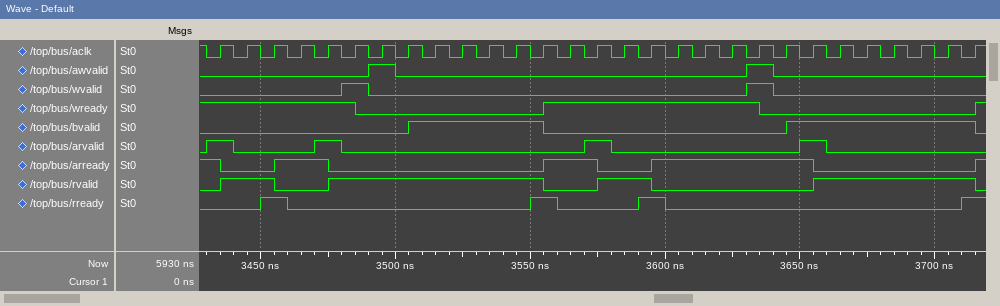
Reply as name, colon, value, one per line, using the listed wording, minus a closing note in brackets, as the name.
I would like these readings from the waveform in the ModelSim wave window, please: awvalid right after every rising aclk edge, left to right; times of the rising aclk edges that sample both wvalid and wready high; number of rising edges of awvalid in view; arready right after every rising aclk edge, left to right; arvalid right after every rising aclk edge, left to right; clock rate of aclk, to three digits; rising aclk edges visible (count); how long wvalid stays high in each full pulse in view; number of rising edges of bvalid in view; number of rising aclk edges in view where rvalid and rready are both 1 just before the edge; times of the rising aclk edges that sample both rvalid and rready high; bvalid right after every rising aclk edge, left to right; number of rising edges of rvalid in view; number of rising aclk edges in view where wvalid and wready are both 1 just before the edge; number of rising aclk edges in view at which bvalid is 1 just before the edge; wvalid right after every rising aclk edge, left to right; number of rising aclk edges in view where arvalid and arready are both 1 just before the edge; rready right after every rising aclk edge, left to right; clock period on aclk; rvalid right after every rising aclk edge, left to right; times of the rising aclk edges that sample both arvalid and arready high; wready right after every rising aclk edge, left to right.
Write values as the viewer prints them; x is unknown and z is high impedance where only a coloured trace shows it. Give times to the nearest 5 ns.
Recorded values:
awvalid right after every rising aclk edge, left to right: 0 0 0 0 0 0 1 0 0 0 0 0 0 0 0 0 0 0 0 0 1 0 0 0 0 0 0 0 0
times of the rising aclk edges that sample both wvalid and wready high: 3485 ns, 3635 ns
number of rising edges of awvalid in view: 2
arready right after every rising aclk edge, left to right: 0 0 1 1 0 0 0 0 0 0 0 0 1 1 0 0 1 1 1 1 1 1 0 0 0 0 0 0 1
arvalid right after every rising aclk edge, left to right: 1 0 0 0 1 0 0 0 0 0 0 0 0 0 1 0 0 0 0 0 0 0 1 0 0 0 0 0 0
clock rate of aclk, to three digits: 100 MHz
rising aclk edges visible: 29
how long wvalid stays high in each full pulse in view: 10 ns, 10 ns
number of rising edges of bvalid in view: 2
number of rising aclk edges in view where rvalid and rready are both 1 just before the edge: 4
times of the rising aclk edges that sample both rvalid and rready high: 3455 ns, 3555 ns, 3595 ns, 3715 ns
bvalid right after every rising aclk edge, left to right: 0 0 0 0 0 0 0 1 1 1 1 1 0 0 0 0 0 0 0 0 0 1 1 1 1 1 1 1 0
number of rising edges of rvalid in view: 4
number of rising aclk edges in view where wvalid and wready are both 1 just before the edge: 2
number of rising aclk edges in view at which bvalid is 1 just before the edge: 12
wvalid right after every rising aclk edge, left to right: 0 0 0 0 0 1 0 0 0 0 0 0 0 0 0 0 0 0 0 0 1 0 0 0 0 0 0 0 0
number of rising aclk edges in view where arvalid and arready are both 1 just before the edge: 4
rready right after every rising aclk edge, left to right: 0 0 1 0 0 0 0 0 0 0 0 0 1 0 0 0 1 0 0 0 0 0 0 0 0 0 0 0 1
clock period on aclk: 10 ns
rvalid right after every rising aclk edge, left to right: 1 1 0 0 1 1 1 1 1 1 1 1 0 0 1 1 0 0 0 0 0 0 1 1 1 1 1 1 0
times of the rising aclk edges that sample both arvalid and arready high: 3435 ns, 3475 ns, 3575 ns, 3655 ns
wready right after every rising aclk edge, left to right: 1 1 1 1 1 0 0 0 0 0 0 0 1 1 1 1 1 1 1 1 0 0 0 0 0 0 0 0 1
